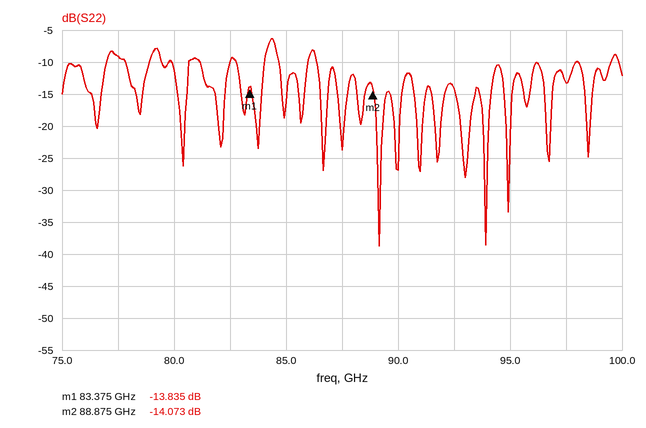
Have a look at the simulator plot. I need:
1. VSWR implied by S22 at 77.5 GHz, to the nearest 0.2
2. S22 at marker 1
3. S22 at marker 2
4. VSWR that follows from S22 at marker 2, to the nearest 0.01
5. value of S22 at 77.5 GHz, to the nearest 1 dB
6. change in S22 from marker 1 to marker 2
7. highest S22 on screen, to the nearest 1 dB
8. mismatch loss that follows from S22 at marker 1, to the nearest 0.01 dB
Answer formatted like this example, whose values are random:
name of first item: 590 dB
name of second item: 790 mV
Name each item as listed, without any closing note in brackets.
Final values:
VSWR implied by S22 at 77.5 GHz, to the nearest 0.2: 2.0
S22 at marker 1: -13.835 dB
S22 at marker 2: -14.073 dB
VSWR that follows from S22 at marker 2, to the nearest 0.01: 1.49
value of S22 at 77.5 GHz, to the nearest 1 dB: -9 dB
change in S22 from marker 1 to marker 2: -0.238 dB
highest S22 on screen, to the nearest 1 dB: -6 dB
mismatch loss that follows from S22 at marker 1, to the nearest 0.01 dB: 0.18 dB
